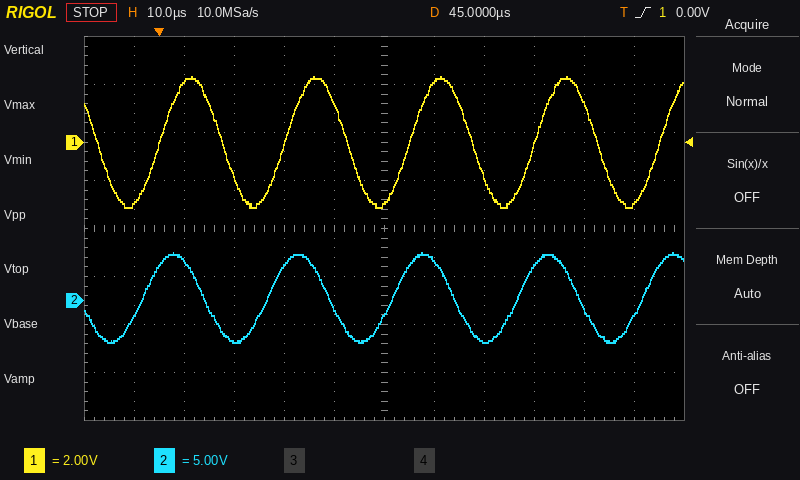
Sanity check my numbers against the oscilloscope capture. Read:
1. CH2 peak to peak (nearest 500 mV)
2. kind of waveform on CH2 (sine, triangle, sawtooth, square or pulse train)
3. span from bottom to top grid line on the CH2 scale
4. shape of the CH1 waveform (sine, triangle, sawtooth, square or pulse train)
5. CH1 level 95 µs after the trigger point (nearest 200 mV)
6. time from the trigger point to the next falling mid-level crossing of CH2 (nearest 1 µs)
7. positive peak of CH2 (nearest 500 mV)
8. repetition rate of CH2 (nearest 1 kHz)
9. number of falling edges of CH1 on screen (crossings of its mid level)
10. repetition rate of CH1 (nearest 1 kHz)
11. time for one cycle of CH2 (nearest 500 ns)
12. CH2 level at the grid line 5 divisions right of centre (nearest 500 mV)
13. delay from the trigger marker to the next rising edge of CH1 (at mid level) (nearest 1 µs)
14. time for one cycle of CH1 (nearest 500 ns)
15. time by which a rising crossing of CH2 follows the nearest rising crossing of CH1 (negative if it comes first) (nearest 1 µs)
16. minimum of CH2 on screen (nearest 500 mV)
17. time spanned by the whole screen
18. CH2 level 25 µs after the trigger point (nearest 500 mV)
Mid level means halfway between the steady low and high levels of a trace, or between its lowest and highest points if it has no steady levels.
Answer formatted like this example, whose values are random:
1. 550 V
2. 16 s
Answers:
1. 9.5 V
2. sine
3. 40 V
4. sine
5. -2.6 V
6. 9 µs
7. 5.0 V
8. 40 kHz
9. 5
10. 40 kHz
11. 25.0 µs
12. -1.5 V
13. 25 µs
14. 25.0 µs
15. -3 µs
16. -4.5 V
17. 120 µs
18. 3.5 V
